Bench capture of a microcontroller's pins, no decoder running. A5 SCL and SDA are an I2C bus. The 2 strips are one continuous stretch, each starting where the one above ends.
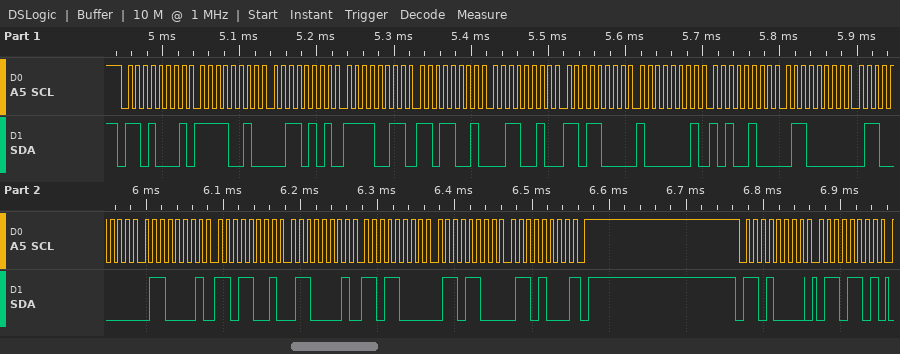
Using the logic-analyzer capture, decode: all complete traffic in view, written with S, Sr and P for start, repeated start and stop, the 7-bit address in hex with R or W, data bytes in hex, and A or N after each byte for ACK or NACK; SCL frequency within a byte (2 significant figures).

S 68R A F2 A 35 A F3 A D9 A 32 A D8 A 81 A A4 A 60 A 60 A 61 A D9 A 61 A D8 A 6C A 68 N P S 68W A 6D A
100 kHz
